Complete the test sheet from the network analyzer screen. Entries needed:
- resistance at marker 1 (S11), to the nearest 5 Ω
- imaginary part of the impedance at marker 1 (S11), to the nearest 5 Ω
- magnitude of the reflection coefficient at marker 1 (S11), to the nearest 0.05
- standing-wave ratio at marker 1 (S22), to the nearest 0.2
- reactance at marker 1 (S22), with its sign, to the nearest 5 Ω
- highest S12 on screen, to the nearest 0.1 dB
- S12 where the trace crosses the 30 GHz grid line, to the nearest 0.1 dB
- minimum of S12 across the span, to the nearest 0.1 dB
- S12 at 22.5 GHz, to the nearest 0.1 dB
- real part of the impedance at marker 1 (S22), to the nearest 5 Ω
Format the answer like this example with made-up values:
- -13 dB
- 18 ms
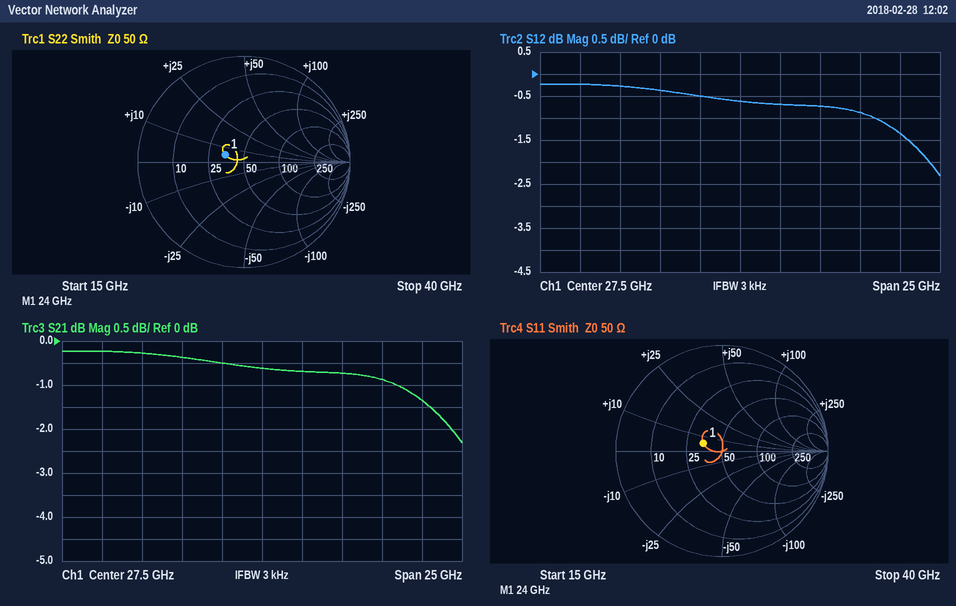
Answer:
- 35 Ω
- +5 Ω
- 0.20
- 1.4
- +5 Ω
- -0.2 dB
- -0.7 dB
- -2.3 dB
- -0.4 dB
- 35 Ω
